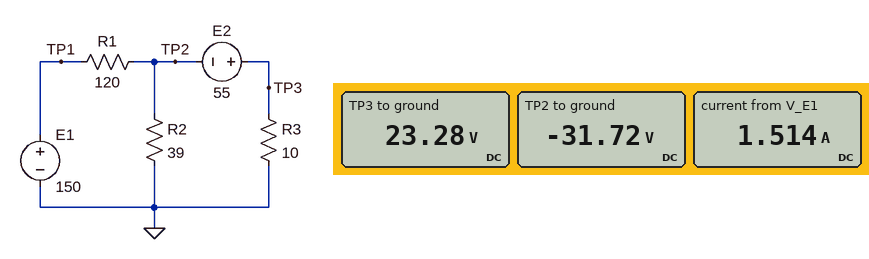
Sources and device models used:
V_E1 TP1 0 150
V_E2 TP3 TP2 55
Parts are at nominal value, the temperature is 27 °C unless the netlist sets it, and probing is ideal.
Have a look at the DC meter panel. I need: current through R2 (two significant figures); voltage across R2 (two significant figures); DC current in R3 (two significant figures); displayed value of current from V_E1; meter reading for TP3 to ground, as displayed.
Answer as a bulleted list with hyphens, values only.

- 810 mA
- 32 V
- 2.3 A
- 1.514 A
- 23.28 V
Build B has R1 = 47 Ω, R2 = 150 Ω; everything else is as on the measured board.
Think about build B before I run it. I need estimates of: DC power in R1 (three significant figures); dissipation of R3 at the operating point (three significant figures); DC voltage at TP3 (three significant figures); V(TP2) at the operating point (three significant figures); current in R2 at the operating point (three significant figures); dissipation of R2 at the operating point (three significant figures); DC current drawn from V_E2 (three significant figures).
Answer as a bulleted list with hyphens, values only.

- 601 W
- 137 W
- 37.0 V
- -18.0 V
- 120 mA
- 2.17 W
- 3.70 A
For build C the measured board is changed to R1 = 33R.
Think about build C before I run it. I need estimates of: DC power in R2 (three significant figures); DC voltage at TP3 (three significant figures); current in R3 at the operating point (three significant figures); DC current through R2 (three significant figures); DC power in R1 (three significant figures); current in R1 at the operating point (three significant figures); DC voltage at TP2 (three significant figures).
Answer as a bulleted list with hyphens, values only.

- 961 mW
- 48.9 V
- 4.89 A
- 157 mA
- 739 W
- 4.73 A
- -6.12 V
